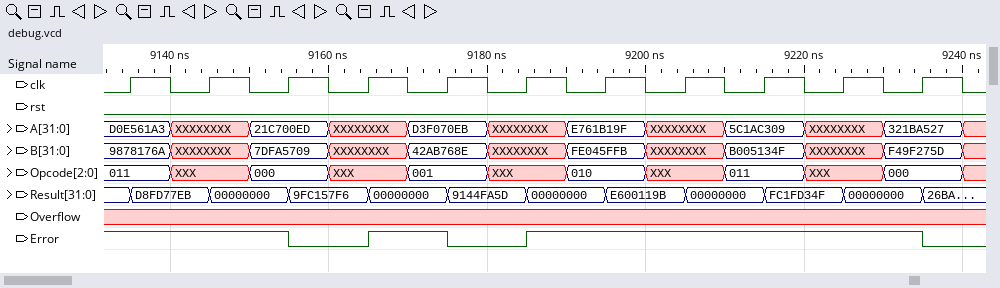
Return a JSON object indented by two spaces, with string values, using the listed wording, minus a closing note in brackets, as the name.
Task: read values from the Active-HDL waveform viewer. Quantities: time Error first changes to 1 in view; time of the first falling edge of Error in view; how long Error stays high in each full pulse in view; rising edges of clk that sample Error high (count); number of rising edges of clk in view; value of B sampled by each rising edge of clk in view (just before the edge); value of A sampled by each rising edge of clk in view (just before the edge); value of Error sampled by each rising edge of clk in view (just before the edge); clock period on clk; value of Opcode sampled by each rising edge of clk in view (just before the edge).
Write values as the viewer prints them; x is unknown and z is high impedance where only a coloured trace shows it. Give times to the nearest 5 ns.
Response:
{
  "time Error first changes to 1 in view": "9165 ns",
  "time of the first falling edge of Error in view": "9155 ns",
  "how long Error stays high in each full pulse in view": "10 ns, 50 ns",
  "rising edges of clk that sample Error high": "9",
  "number of rising edges of clk in view": "11",
  "value of B sampled by each rising edge of clk in view": "9878176A, XXXXXXXX, 7DFA5709, XXXXXXXX, 42AB768E, XXXXXXXX, FE045FFB, XXXXXXXX, B005134F, XXXXXXXX, F49F275D",
  "value of A sampled by each rising edge of clk in view": "D0E561A3, XXXXXXXX, 21C700ED, XXXXXXXX, D3F070EB, XXXXXXXX, E761B19F, XXXXXXXX, 5C1AC309, XXXXXXXX, 321BA527",
  "value of Error sampled by each rising edge of clk in view": "1 1 1 0 1 0 1 1 1 1 1",
  "clock period on clk": "10 ns",
  "value of Opcode sampled by each rising edge of clk in view": "011, XXX, 000, XXX, 001, XXX, 010, XXX, 011, XXX, 000"
}
